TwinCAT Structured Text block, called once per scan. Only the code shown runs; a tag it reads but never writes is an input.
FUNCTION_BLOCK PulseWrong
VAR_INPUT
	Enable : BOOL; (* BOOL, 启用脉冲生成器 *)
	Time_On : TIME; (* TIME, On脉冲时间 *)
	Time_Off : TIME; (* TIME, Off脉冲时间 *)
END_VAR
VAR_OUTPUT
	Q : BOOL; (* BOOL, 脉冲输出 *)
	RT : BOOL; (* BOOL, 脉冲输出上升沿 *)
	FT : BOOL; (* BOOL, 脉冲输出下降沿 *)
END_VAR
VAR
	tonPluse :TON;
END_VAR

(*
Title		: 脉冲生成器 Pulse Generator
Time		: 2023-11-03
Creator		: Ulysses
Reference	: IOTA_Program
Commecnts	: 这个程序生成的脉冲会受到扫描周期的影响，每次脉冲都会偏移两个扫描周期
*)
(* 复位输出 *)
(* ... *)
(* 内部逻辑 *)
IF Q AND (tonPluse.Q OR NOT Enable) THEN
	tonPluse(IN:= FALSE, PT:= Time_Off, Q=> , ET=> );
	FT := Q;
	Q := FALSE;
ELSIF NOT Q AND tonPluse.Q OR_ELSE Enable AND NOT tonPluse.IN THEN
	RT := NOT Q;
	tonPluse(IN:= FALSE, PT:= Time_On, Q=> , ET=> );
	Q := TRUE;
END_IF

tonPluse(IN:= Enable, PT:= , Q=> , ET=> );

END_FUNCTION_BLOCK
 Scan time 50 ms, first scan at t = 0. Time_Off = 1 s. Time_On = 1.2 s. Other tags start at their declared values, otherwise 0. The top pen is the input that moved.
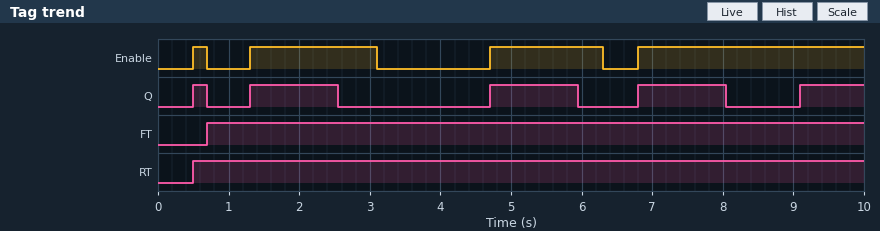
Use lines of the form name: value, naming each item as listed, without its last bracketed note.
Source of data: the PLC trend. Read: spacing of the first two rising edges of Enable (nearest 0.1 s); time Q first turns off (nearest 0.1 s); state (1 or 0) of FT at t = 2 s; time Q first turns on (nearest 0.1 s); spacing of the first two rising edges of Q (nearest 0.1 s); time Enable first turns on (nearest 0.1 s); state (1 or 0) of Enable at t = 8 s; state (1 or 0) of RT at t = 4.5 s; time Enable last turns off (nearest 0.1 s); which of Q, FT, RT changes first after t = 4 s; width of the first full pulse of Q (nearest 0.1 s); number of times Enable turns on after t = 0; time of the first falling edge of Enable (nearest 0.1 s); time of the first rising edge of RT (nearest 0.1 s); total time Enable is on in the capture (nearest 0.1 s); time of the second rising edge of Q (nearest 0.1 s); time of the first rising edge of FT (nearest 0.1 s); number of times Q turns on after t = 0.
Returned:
spacing of the first two rising edges of Enable: 0.8 s
time Q first turns off: 0.7 s
state (1 or 0) of FT at t = 2 s: 1
time Q first turns on: 0.5 s
spacing of the first two rising edges of Q: 0.8 s
time Enable first turns on: 0.5 s
state (1 or 0) of Enable at t = 8 s: 1
state (1 or 0) of RT at t = 4.5 s: 1
time Enable last turns off: 6.3 s
which of Q, FT, RT changes first after t = 4 s: Q
width of the first full pulse of Q: 0.2 s
number of times Enable turns on after t = 0: 4
time of the first falling edge of Enable: 0.7 s
time of the first rising edge of RT: 0.5 s
total time Enable is on in the capture: 6.8 s
time of the second rising edge of Q: 1.3 s
time of the first rising edge of FT: 0.7 s
number of times Q turns on after t = 0: 5
